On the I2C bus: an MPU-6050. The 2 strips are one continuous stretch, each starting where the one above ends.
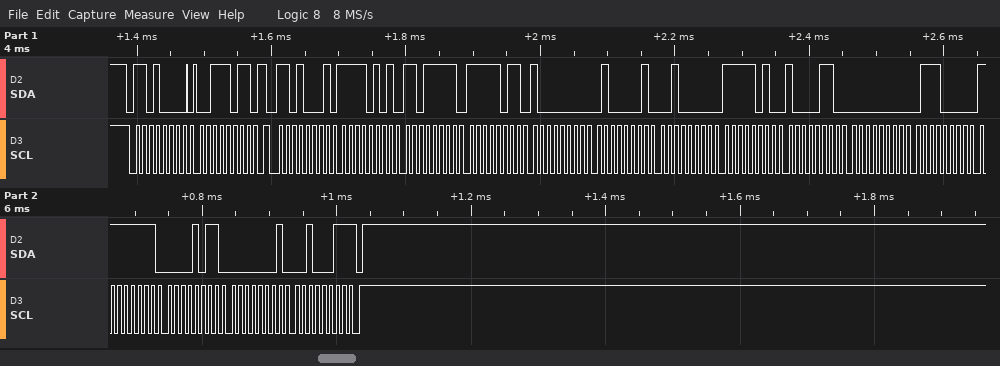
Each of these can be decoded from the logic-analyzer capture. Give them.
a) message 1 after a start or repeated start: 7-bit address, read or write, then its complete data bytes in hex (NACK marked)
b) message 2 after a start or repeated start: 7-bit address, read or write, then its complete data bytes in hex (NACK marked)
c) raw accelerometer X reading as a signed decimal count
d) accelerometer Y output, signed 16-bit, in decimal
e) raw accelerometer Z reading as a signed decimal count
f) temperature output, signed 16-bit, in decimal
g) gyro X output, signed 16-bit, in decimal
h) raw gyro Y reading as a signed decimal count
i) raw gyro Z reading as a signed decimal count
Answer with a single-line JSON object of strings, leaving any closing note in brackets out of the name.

{"message 1 after a start or repeated start: 7-bit address, read or write, then its complete data bytes in hex": "0x68 write: 3B", "message 2 after a start or repeated start: 7-bit address, read or write, then its complete data bytes in hex": "0x68 read: F5 DF FB 80 41 20 FA 86 00 70 FF 0B 01 23 NACK", "raw accelerometer X reading as a signed decimal count": "-2593", "accelerometer Y output, signed 16-bit, in decimal": "-1152", "raw accelerometer Z reading as a signed decimal count": "16672", "temperature output, signed 16-bit, in decimal": "-1402", "gyro X output, signed 16-bit, in decimal": "112", "raw gyro Y reading as a signed decimal count": "-245", "raw gyro Z reading as a signed decimal count": "291"}
